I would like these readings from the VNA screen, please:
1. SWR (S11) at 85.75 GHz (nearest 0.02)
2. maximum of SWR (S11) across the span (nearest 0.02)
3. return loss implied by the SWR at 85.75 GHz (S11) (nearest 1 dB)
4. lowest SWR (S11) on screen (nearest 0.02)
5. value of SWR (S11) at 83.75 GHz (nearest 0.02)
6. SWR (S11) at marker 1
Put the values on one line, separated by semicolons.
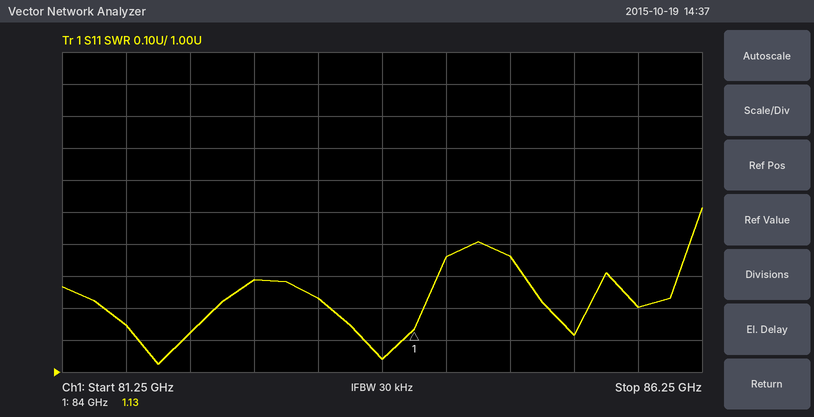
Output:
1.20; 1.52; 21 dB; 1.02; 1.04; 1.13
